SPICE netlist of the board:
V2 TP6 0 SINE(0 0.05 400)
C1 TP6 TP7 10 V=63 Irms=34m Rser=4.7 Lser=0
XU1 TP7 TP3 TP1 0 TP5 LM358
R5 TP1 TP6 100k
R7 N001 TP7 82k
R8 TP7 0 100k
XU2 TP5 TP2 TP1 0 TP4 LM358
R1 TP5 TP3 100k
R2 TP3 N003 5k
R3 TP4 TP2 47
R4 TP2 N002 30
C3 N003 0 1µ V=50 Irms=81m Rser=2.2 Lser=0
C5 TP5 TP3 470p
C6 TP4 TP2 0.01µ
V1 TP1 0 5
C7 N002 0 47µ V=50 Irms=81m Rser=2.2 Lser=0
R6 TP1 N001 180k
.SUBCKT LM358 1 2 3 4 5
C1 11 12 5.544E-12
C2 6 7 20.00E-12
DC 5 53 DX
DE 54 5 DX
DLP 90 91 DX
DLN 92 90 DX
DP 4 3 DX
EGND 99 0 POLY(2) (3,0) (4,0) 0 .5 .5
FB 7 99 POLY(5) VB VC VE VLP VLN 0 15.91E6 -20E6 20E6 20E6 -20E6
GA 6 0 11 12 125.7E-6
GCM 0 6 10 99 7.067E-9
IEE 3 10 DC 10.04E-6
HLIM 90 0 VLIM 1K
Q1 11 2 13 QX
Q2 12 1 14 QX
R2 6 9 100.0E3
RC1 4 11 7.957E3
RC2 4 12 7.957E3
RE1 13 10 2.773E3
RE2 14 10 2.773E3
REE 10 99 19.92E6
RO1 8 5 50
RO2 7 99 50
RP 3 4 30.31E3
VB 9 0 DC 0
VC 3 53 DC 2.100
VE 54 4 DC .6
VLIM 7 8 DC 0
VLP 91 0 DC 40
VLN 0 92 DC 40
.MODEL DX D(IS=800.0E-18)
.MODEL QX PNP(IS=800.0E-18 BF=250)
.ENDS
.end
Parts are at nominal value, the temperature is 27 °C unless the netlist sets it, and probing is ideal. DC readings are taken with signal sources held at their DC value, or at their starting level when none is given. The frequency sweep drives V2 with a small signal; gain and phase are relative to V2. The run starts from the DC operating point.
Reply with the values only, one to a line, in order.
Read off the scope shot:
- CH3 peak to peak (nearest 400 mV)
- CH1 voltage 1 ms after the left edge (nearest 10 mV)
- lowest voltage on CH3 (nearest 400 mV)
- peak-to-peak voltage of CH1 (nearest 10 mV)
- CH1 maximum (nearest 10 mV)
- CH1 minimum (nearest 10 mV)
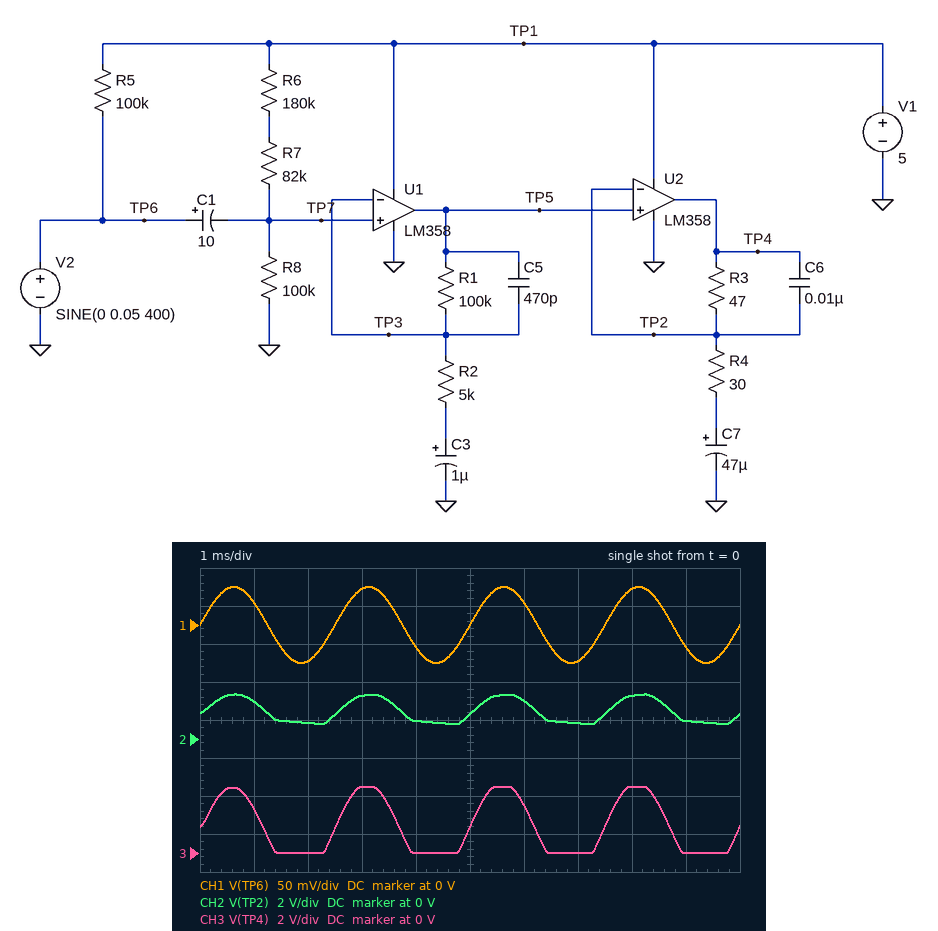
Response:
3.6 V
30 mV
0 V
100 mV
50 mV
-50 mV
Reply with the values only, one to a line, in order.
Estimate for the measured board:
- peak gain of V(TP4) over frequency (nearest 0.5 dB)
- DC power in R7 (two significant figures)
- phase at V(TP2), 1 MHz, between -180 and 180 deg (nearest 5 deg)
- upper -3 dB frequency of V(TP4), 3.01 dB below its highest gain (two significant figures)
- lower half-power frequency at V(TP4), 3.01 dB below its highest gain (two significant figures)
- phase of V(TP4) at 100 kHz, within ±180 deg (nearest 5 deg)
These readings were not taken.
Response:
34.0 dB
16 µW
-160 deg
3.4 kHz
92 Hz
-70 deg
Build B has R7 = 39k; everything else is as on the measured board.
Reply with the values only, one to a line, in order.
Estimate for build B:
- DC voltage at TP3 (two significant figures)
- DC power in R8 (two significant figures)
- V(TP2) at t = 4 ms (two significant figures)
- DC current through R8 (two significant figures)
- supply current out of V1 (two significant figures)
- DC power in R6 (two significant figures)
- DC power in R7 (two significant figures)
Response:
1.6 V
25 µW
1.0 V
16 µA
420 µA
44 µW
9.6 µW
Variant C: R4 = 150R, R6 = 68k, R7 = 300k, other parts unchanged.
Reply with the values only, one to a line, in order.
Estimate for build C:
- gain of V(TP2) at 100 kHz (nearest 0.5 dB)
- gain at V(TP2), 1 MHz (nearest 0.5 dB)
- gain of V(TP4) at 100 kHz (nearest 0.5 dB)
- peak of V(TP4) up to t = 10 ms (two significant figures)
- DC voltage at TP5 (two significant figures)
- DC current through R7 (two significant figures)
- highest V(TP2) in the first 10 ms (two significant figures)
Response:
1.0 dB
-4.5 dB
3.5 dB
2.4 V
1.1 V
11 µA
2.1 V
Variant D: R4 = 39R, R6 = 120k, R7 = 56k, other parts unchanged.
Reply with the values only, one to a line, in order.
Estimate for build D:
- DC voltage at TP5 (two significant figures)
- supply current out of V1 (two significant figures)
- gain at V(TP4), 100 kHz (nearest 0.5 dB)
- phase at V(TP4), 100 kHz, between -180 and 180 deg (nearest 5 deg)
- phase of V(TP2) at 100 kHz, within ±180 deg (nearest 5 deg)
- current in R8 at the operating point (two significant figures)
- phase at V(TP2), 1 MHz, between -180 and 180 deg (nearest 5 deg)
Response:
1.8 V
420 µA
7.0 dB
-65 deg
-55 deg
18 µA
-155 deg
